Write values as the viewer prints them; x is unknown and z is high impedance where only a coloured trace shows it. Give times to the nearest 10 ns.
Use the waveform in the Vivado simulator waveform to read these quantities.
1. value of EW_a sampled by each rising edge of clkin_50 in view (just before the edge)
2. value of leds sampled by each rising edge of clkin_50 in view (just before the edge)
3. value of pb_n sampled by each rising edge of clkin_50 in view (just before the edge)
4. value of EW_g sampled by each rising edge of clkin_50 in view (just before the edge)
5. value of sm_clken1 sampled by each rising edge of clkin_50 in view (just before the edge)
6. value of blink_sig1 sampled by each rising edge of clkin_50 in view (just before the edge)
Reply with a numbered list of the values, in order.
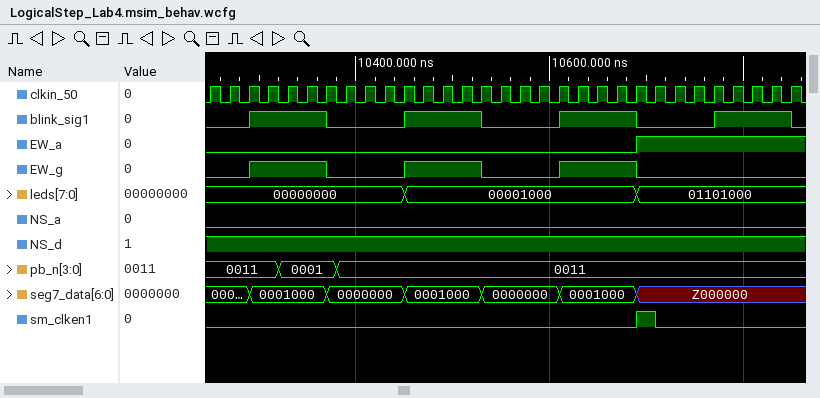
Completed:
1. 0 0 0 0 0 0 0 0 0 0 0 0 0 0 0 0 0 0 0 0 0 0 0 1 1 1 1 1 1 1 1
2. 00000000, 00000000, 00000000, 00000000, 00000000, 00000000, 00000000, 00000000, 00000000, 00000000, 00000000, 00001000, 00001000, 00001000, 00001000, 00001000, 00001000, 00001000, 00001000, 00001000, 00001000, 00001000, 00001000, 01101000, 01101000, 01101000, 01101000, 01101000, 01101000, 01101000, 01101000
3. 0011, 0011, 0011, 0011, 0001, 0001, 0001, 0011, 0011, 0011, 0011, 0011, 0011, 0011, 0011, 0011, 0011, 0011, 0011, 0011, 0011, 0011, 0011, 0011, 0011, 0011, 0011, 0011, 0011, 0011, 0011
4. 0 0 0 1 1 1 1 0 0 0 0 1 1 1 1 0 0 0 0 1 1 1 1 0 0 0 0 0 0 0 0
5. 0 0 0 0 0 0 0 0 0 0 0 0 0 0 0 0 0 0 0 0 0 0 0 1 0 0 0 0 0 0 0
6. 0 0 0 1 1 1 1 0 0 0 0 1 1 1 1 0 0 0 0 1 1 1 1 0 0 0 0 1 1 1 1
